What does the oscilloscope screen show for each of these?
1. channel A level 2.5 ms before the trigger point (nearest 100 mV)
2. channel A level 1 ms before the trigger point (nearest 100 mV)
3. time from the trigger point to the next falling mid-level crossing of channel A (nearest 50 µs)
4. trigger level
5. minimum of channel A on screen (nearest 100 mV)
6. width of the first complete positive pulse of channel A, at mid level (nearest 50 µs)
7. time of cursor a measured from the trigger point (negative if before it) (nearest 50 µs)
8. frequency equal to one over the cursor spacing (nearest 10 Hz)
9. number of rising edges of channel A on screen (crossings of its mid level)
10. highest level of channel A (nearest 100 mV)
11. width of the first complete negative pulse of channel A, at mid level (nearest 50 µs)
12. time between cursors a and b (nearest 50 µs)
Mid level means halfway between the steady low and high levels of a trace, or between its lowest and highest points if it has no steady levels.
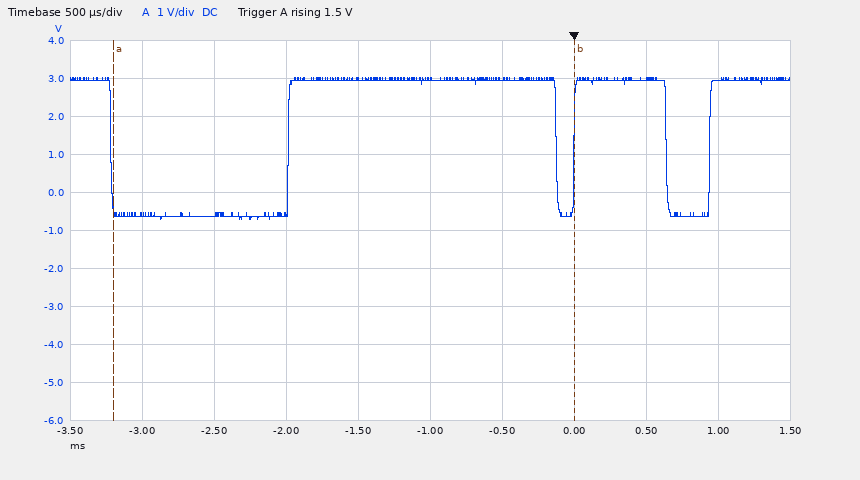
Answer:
-600 mV
3.0 V
650 µs
1.5 V
-700 mV
1.85 ms
-3.20 ms
310 Hz
3
3.0 V
1.25 ms
3.20 ms
